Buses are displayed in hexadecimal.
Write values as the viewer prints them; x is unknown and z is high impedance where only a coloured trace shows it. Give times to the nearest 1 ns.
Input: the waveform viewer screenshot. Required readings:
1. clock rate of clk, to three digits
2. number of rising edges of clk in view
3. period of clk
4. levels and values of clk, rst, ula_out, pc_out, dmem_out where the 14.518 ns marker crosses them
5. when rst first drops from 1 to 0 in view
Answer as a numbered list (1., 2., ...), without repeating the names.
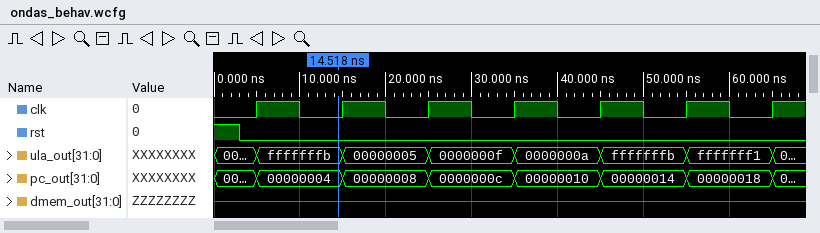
1. 100 MHz
2. 7
3. 10 ns
4. clk=0, rst=0, ula_out=fffffffb, pc_out=00000004, dmem_out=z
5. 3 ns
